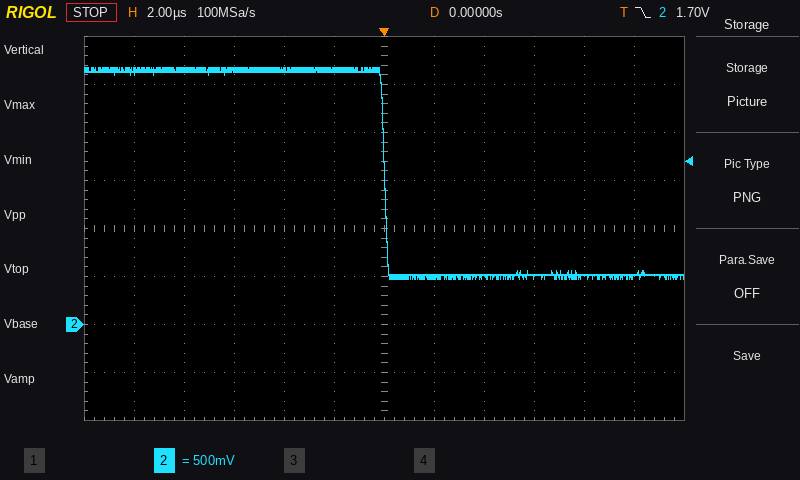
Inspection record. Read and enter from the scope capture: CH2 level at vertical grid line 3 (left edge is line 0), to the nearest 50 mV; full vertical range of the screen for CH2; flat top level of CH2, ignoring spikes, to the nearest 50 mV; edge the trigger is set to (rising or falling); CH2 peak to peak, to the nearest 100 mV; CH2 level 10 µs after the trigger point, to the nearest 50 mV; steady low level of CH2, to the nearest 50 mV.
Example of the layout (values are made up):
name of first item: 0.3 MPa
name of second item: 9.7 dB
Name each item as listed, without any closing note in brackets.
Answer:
CH2 level at vertical grid line 3 (left edge is line 0), to the nearest 50 mV: 2.65 V
full vertical range of the screen for CH2: 4 V
flat top level of CH2, ignoring spikes, to the nearest 50 mV: 2.65 V
edge the trigger is set to: falling
CH2 peak to peak, to the nearest 100 mV: 2.20 V
CH2 level 10 µs after the trigger point, to the nearest 50 mV: 500 mV
steady low level of CH2, to the nearest 50 mV: 500 mV
